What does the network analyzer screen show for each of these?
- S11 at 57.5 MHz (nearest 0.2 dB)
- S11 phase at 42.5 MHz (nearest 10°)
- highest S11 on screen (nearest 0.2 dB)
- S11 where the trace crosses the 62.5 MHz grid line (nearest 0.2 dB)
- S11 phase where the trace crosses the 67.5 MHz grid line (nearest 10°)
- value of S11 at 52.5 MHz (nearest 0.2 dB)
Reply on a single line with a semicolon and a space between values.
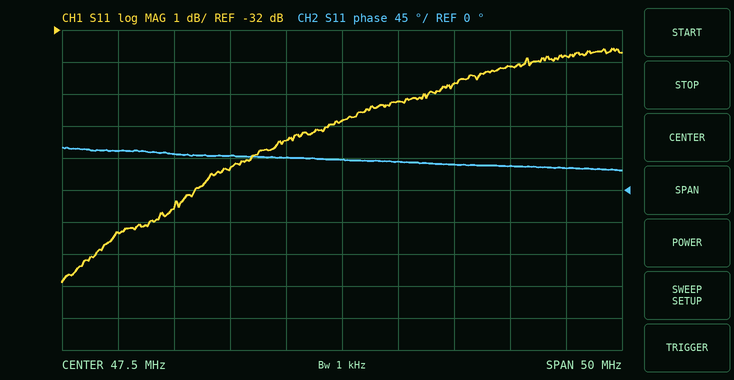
-33.6 dB; 50°; -32.6 dB; -33.2 dB; 30°; -34.2 dB
